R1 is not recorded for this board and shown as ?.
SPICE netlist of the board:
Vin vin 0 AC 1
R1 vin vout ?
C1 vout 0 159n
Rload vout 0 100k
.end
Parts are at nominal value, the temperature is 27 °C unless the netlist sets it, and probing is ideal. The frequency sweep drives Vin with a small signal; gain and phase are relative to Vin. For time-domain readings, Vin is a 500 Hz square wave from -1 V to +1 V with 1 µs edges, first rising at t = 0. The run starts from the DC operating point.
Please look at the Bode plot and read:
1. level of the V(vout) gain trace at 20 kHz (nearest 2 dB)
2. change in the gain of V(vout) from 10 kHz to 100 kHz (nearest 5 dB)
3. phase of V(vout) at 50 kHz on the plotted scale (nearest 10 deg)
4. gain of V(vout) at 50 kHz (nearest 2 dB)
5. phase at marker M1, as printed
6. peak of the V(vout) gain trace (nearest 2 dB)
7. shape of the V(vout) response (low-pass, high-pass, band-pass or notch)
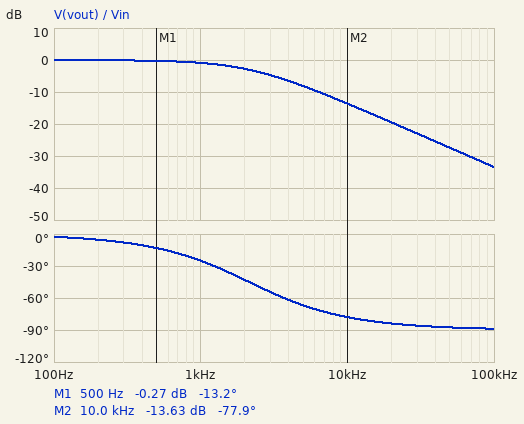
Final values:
-20 dB
-20 dB
-90 deg
-28 dB
-13.2 deg
0 dB
low-pass
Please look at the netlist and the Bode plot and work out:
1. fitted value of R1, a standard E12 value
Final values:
470 Ω
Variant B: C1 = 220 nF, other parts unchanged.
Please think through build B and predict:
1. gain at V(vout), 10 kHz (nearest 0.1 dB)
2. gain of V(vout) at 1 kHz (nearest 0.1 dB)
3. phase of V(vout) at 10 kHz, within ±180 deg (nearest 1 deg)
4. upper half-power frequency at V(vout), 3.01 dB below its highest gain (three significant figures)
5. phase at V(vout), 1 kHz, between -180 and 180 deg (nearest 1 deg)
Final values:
-16.4 dB
-1.6 dB
-81 deg
1.55 kHz
-33 deg
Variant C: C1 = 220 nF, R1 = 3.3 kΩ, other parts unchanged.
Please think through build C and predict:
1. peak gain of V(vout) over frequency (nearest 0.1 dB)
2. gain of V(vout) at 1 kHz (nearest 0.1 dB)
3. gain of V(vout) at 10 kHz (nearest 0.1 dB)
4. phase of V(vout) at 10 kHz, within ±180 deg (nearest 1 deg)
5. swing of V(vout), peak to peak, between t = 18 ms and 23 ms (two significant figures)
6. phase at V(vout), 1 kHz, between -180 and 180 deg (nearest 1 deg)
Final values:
-0.3 dB
-13.4 dB
-33.2 dB
-89 deg
1.2 V
-77 deg
